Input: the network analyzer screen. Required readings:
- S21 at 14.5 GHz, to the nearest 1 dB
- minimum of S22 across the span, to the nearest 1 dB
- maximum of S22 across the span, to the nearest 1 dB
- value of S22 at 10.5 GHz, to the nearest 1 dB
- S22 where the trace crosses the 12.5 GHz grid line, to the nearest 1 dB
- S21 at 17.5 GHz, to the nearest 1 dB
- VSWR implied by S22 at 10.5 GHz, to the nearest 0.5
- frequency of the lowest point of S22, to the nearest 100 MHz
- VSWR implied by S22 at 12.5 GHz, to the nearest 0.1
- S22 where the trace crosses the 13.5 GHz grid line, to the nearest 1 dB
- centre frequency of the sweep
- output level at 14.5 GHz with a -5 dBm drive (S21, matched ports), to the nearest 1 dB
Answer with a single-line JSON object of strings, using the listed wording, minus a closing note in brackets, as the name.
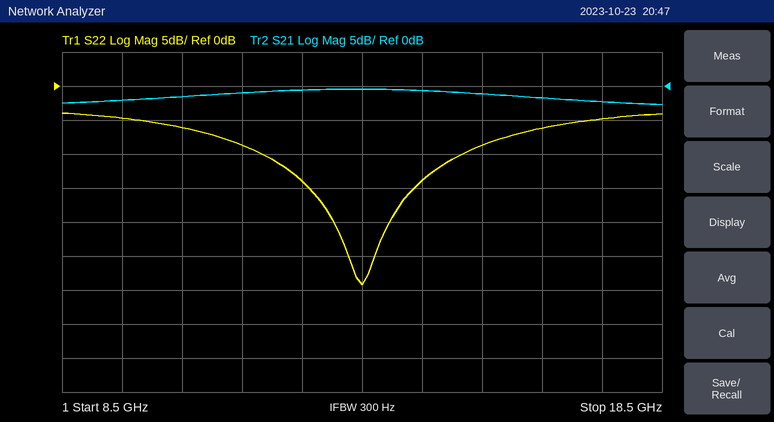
{"S21 at 14.5 GHz, to the nearest 1 dB": "-1 dB", "minimum of S22 across the span, to the nearest 1 dB": "-29 dB", "maximum of S22 across the span, to the nearest 1 dB": "-4 dB", "value of S22 at 10.5 GHz, to the nearest 1 dB": "-6 dB", "S22 where the trace crosses the 12.5 GHz grid line, to the nearest 1 dB": "-14 dB", "S21 at 17.5 GHz, to the nearest 1 dB": "-2 dB", "VSWR implied by S22 at 10.5 GHz, to the nearest 0.5": "3.0", "frequency of the lowest point of S22, to the nearest 100 MHz": "13.5 GHz", "VSWR implied by S22 at 12.5 GHz, to the nearest 0.1": "1.5", "S22 where the trace crosses the 13.5 GHz grid line, to the nearest 1 dB": "-29 dB", "centre frequency of the sweep": "13.5 GHz", "output level at 14.5 GHz with a -5 dBm drive (S21, matched ports), to the nearest 1 dB": "-6 dBm"}
